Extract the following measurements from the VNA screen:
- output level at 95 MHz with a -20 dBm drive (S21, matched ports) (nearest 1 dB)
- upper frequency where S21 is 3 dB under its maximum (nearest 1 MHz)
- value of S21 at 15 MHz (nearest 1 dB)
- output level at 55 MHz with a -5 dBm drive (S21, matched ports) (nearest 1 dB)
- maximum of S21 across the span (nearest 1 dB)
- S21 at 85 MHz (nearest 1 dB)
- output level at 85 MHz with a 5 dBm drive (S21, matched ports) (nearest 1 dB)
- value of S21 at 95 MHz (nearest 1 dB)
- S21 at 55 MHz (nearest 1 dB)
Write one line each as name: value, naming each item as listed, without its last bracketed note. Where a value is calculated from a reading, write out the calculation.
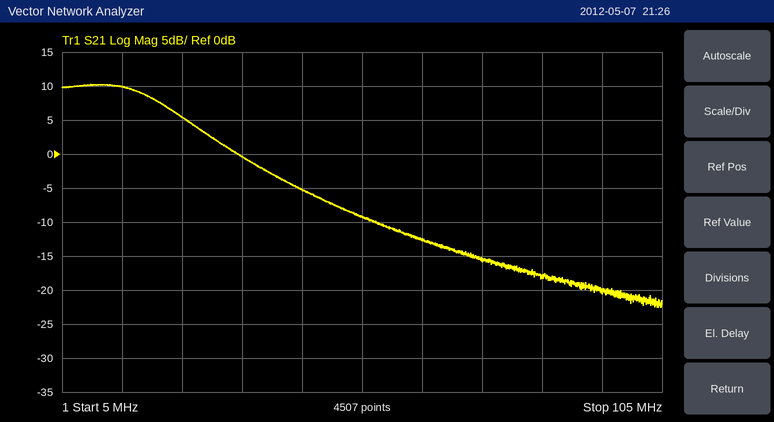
output level at 95 MHz with a -20 dBm drive (S21, matched ports): -20 dBm + (-20 dB) = -40 dBm
upper frequency where S21 is 3 dB under its maximum: 22 MHz
value of S21 at 15 MHz: 10 dB
output level at 55 MHz with a -5 dBm drive (S21, matched ports): -5 dBm + (-9 dB) = -14 dBm
maximum of S21 across the span: 10 dB
S21 at 85 MHz: -18 dB
output level at 85 MHz with a 5 dBm drive (S21, matched ports): 5 dBm + (-18 dB) = -13 dBm
value of S21 at 95 MHz: -20 dB
S21 at 55 MHz: -9 dB
